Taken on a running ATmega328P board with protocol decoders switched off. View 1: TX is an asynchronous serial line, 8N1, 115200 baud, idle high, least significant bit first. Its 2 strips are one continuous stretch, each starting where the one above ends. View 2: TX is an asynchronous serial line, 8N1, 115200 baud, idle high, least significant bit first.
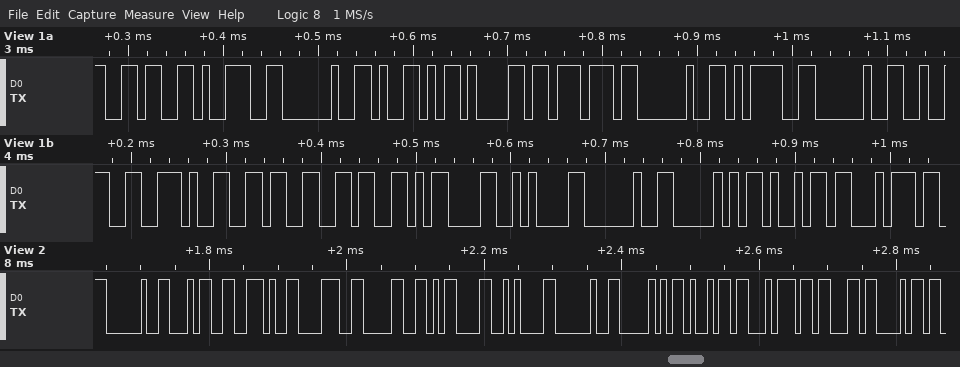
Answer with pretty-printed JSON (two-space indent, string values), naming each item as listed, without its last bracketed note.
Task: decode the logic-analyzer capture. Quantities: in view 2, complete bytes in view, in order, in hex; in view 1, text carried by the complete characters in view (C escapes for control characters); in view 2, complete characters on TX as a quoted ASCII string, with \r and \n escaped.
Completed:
{
  "in view 2, complete bytes in view, in order, in hex": "0x20 0x34 0x2E 0x38 0x30 0x0D 0x0A 0x20 0x50 0x69 0x74 0x63 0x68",
  "in view 1, text carried by the complete characters in view": "\"69 Yaw = 2.66\\r\\n Pit\"",
  "in view 2, complete characters on TX as a quoted ASCII string, with \\r and \\n escaped": "\" 4.80\\r\\n Pitch\""
}
